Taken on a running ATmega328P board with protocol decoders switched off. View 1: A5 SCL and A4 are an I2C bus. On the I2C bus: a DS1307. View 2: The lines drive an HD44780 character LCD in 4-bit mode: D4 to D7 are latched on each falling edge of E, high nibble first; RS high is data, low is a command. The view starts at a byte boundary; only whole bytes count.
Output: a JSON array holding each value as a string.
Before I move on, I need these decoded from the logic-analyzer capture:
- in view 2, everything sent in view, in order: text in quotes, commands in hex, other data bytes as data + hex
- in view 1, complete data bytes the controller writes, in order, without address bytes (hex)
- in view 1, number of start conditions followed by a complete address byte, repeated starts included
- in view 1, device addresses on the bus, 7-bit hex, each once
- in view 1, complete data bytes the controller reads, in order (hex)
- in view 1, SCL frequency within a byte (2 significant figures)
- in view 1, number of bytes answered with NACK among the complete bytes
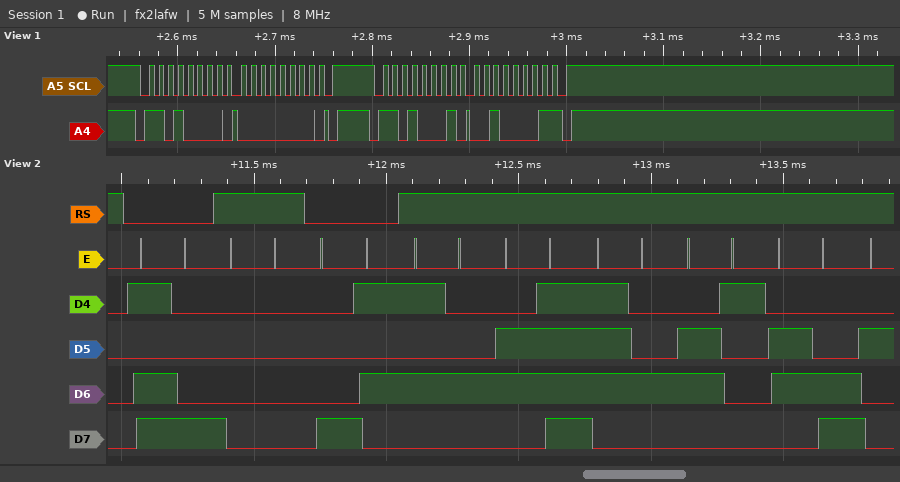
["0xD8 data 00 0x85 \"Total\"", "00", "2", "0x68", "21", "100 kHz", "1"]
